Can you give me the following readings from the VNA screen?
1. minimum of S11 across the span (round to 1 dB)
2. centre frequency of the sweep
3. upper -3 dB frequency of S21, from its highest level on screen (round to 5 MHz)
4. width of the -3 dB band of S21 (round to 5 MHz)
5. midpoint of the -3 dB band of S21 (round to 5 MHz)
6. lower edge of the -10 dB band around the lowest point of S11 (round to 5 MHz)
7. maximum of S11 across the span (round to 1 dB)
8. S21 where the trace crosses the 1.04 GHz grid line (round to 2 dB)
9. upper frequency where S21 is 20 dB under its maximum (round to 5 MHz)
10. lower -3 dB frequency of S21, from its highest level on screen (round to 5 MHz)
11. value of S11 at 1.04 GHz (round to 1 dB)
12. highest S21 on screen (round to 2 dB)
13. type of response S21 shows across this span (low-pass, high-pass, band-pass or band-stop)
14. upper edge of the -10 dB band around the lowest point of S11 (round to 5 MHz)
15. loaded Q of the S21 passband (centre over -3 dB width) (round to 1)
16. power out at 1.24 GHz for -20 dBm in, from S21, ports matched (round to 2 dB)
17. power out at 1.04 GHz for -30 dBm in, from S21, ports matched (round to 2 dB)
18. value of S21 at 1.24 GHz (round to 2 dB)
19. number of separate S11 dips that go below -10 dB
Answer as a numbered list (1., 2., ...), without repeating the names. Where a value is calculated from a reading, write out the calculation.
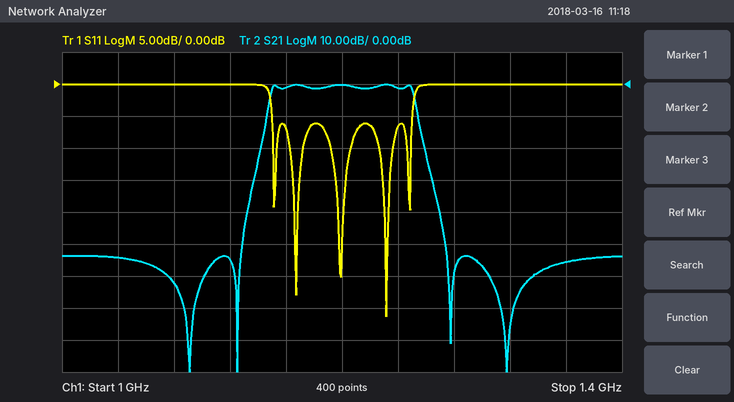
1. -36 dB
2. 1.2 GHz
3. 1.250 GHz
4. 1.250 GHz − 1.150 GHz = 100 MHz
5. 1.200 GHz
6. 1.225 GHz
7. 0 dB
8. -54 dB
9. 1.260 GHz
10. 1.150 GHz
11. 0 dB
12. 0 dB
13. band-pass
14. 1.235 GHz
15. 1.2 GHz / 100 MHz ≈ 12
16. -20 dBm + (-2 dB) = -22 dBm
17. -30 dBm + (-54 dB) = -84 dBm
18. -2 dB
19. 5
